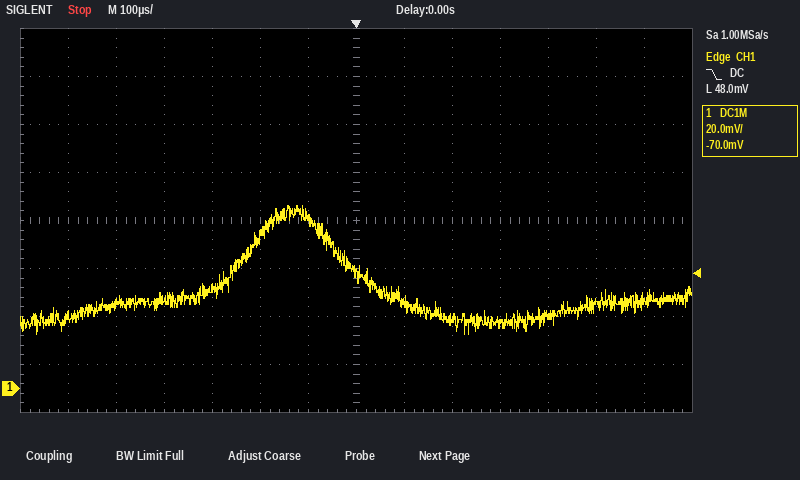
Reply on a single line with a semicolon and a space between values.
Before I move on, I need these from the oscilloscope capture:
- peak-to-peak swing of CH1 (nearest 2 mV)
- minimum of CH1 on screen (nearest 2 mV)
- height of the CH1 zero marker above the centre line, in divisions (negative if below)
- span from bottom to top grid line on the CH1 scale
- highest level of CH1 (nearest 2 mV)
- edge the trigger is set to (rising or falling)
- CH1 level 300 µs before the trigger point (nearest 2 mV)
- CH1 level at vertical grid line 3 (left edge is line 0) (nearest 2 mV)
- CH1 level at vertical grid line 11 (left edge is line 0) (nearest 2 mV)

54 mV; 22 mV; -3.5 div; 160 mV; 76 mV; falling; 42 mV; 36 mV; 30 mV
